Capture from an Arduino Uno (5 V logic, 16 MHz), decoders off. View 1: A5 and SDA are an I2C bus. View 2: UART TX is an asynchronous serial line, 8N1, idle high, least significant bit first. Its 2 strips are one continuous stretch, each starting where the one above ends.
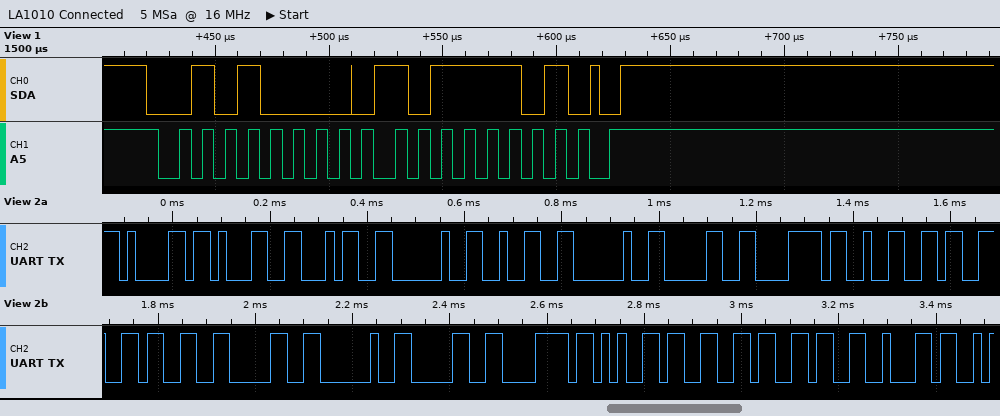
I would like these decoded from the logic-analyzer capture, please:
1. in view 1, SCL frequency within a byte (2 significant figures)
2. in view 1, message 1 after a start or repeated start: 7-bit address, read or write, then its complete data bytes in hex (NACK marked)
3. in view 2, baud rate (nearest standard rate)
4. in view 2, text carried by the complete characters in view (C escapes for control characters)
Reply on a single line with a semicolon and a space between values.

100 kHz; 0x28 write: BD; 57600 baud; "a14 2 0x2330 0xef6b"
